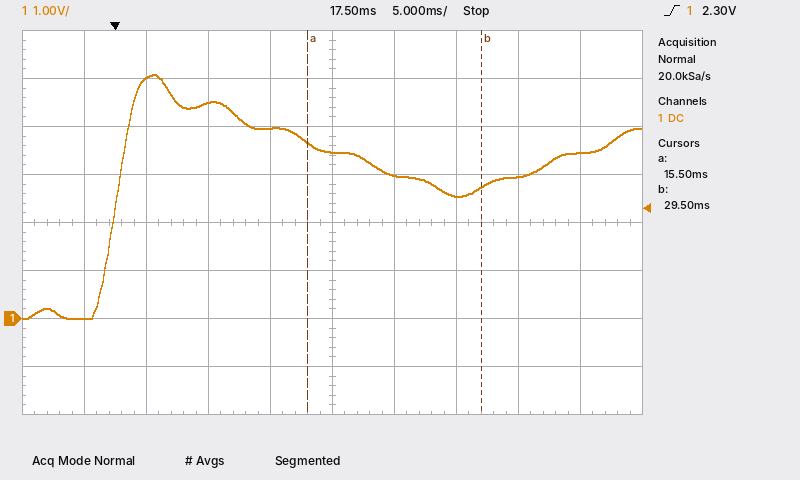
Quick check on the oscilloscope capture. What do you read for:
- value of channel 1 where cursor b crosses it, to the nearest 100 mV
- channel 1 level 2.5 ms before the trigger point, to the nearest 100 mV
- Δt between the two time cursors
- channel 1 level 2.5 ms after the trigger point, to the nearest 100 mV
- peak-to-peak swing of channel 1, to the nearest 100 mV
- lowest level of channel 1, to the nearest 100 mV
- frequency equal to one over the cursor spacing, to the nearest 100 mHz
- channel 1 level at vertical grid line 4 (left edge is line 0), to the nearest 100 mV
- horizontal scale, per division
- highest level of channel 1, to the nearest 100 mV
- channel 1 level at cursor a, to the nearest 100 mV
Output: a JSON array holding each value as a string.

["2.7 V", "0.0 V", "14.0 ms", "5.0 V", "5.1 V", "0.0 V", "71.4 Hz", "4.0 V", "5 ms", "5.1 V", "3.7 V"]
